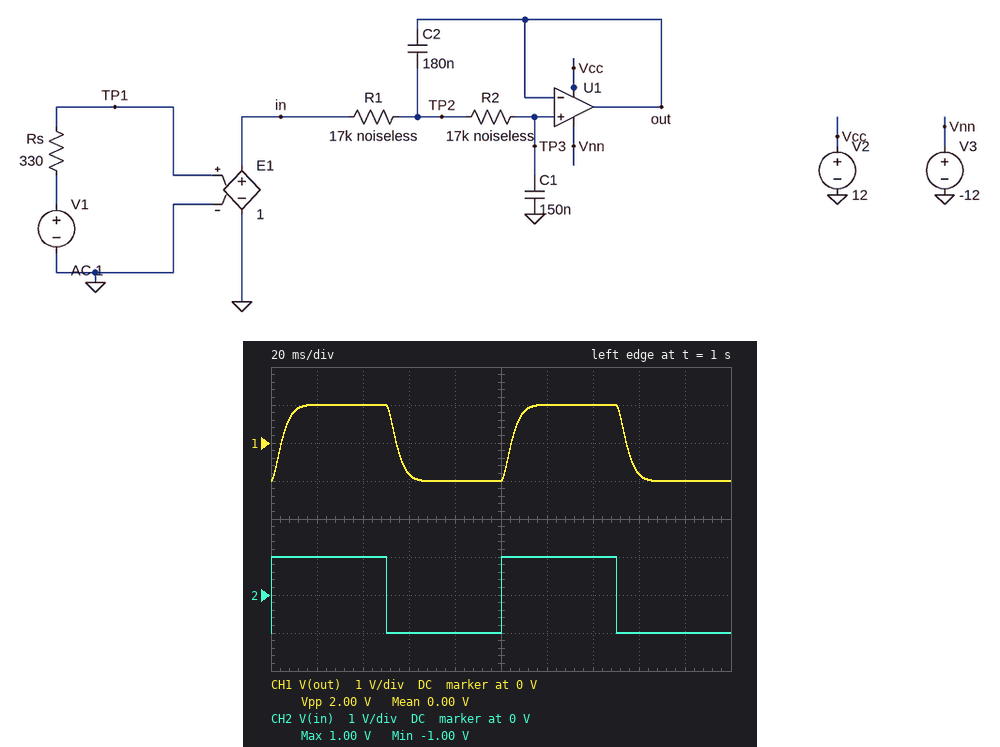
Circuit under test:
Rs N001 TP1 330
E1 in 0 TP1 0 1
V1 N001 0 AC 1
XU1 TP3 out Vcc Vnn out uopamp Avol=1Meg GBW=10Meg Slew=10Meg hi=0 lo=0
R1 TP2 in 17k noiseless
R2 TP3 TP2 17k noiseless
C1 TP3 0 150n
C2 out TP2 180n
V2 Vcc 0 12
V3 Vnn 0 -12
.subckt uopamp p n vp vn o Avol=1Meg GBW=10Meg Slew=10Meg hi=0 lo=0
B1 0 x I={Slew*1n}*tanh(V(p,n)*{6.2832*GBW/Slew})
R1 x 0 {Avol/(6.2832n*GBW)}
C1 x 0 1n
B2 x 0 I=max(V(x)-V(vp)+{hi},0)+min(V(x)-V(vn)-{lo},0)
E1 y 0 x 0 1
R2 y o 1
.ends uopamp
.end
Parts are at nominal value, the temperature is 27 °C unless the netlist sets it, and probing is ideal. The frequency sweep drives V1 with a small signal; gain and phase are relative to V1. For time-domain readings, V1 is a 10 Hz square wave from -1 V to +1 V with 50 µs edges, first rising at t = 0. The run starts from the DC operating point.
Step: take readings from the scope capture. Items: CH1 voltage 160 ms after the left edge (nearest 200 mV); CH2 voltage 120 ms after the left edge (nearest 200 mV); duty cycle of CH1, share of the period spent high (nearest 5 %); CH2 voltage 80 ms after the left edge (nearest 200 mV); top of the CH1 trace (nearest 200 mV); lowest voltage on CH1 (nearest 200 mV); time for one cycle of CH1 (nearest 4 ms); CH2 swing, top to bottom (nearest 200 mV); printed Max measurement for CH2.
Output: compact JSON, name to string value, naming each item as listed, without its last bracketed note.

{"CH1 voltage 160 ms after the left edge": "-800 mV", "CH2 voltage 120 ms after the left edge": "1.0 V", "duty cycle of CH1, share of the period spent high": "50 %", "CH2 voltage 80 ms after the left edge": "-1.0 V", "top of the CH1 trace": "1.0 V", "lowest voltage on CH1": "-1.0 V", "time for one cycle of CH1": "100 ms", "CH2 swing, top to bottom": "2.0 V", "printed Max measurement for CH2": "1.00 V"}
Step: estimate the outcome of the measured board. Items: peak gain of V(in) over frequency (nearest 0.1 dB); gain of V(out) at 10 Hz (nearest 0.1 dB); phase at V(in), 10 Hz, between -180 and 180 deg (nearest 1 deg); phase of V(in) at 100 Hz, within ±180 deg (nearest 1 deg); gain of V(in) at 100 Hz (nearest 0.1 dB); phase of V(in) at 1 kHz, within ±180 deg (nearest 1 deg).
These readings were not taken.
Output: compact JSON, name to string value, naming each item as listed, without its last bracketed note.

{"peak gain of V(in) over frequency": "0 dB", "gain of V(out) at 10 Hz": "-0.2 dB", "phase at V(in), 10 Hz, between -180 and 180 deg": "0 deg", "phase of V(in) at 100 Hz, within ±180 deg": "0 deg", "gain of V(in) at 100 Hz": "0 dB", "phase of V(in) at 1 kHz, within ±180 deg": "0 deg"}
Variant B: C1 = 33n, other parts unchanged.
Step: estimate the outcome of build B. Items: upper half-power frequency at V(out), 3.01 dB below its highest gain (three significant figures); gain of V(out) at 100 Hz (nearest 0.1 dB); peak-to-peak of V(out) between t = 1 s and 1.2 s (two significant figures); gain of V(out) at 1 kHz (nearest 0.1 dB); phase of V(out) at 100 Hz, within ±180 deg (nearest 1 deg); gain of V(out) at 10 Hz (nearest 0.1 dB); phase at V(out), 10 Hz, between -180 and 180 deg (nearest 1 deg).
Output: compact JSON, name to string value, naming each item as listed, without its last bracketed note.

{"upper half-power frequency at V(out), 3.01 dB below its highest gain": "144 Hz", "gain of V(out) at 100 Hz": "2.2 dB", "peak-to-peak of V(out) between t = 1 s and 1.2 s": "2.9 V", "gain of V(out) at 1 kHz": "-36.5 dB", "phase of V(out) at 100 Hz, within ±180 deg": "-65 deg", "gain of V(out) at 10 Hz": "0 dB", "phase at V(out), 10 Hz, between -180 and 180 deg": "-4 deg"}
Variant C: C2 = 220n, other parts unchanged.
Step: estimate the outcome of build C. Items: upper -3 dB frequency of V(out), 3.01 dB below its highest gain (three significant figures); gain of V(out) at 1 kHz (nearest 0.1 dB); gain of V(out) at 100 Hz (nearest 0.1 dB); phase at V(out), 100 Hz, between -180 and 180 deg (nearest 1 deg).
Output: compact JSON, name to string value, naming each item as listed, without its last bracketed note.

{"upper -3 dB frequency of V(out), 3.01 dB below its highest gain": "43.1 Hz", "gain of V(out) at 1 kHz": "-51.5 dB", "gain of V(out) at 100 Hz": "-12.5 dB", "phase at V(out), 100 Hz, between -180 and 180 deg": "-131 deg"}
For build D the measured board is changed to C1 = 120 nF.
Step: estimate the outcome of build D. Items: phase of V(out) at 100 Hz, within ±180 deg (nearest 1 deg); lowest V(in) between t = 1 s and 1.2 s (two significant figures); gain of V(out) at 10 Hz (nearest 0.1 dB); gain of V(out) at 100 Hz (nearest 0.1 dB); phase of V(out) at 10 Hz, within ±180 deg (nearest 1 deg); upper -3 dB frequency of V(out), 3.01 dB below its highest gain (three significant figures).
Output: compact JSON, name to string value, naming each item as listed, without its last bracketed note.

{"phase of V(out) at 100 Hz, within ±180 deg": "-120 deg", "lowest V(in) between t = 1 s and 1.2 s": "-1.0 V", "gain of V(out) at 10 Hz": "-0.1 dB", "gain of V(out) at 100 Hz": "-9.4 dB", "phase of V(out) at 10 Hz, within ±180 deg": "-15 deg", "upper -3 dB frequency of V(out), 3.01 dB below its highest gain": "54.1 Hz"}
